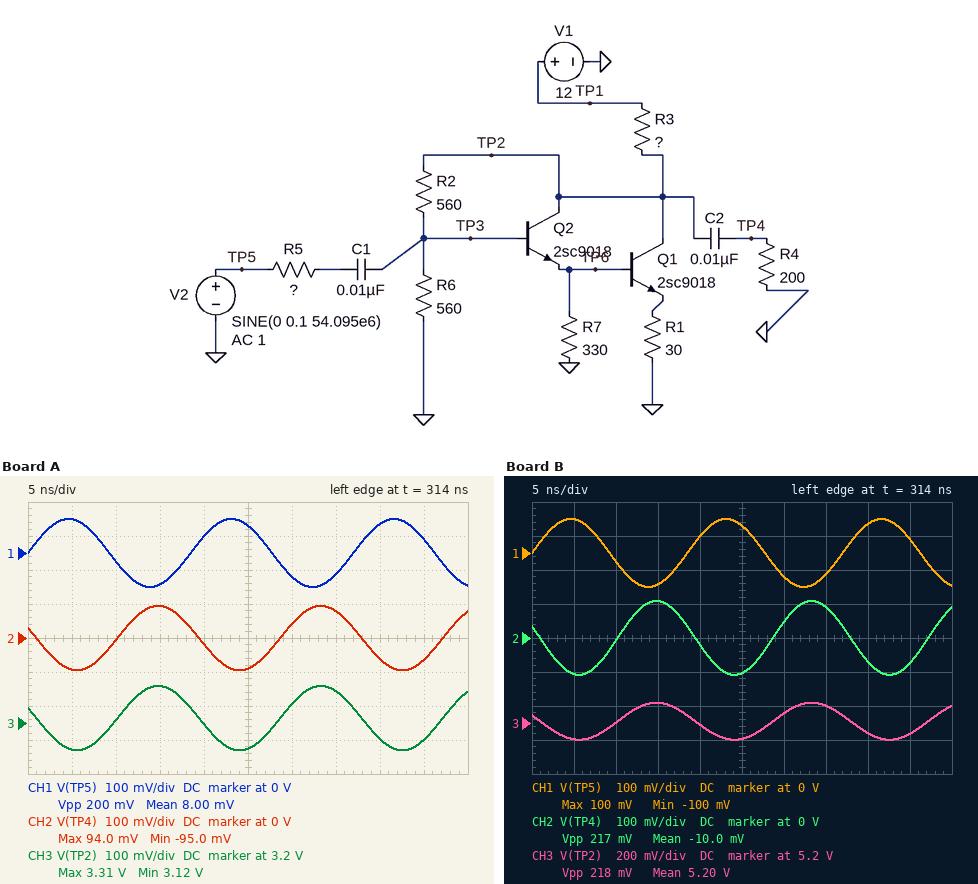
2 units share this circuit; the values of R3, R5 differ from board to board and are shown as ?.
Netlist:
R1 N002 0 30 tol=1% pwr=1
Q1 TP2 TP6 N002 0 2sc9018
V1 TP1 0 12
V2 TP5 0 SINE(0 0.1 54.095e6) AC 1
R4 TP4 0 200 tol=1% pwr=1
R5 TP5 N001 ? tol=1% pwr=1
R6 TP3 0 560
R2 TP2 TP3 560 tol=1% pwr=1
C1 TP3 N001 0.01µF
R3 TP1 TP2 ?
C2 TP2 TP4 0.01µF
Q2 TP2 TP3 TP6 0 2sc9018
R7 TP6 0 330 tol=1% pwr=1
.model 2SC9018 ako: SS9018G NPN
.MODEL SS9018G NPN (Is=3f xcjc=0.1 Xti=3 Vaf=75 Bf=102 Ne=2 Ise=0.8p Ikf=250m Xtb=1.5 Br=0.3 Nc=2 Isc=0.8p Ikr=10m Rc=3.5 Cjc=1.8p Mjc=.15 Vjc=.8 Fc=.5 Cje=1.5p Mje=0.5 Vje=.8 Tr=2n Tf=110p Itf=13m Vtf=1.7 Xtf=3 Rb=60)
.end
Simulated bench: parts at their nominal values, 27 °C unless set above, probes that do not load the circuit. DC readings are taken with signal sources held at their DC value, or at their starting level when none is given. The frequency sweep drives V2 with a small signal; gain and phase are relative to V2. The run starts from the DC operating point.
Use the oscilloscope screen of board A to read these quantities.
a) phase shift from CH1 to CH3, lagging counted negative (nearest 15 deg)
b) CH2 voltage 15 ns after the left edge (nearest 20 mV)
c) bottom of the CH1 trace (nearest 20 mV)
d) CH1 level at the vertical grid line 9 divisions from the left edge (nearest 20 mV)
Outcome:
165 deg
100 mV
-100 mV
40 mV
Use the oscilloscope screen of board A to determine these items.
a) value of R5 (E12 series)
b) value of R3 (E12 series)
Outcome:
270 Ω
820 Ω
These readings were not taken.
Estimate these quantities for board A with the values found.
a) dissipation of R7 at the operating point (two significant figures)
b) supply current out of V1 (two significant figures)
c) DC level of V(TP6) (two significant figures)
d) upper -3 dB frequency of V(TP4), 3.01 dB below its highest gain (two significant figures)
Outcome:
2.4 mW
11 mA
890 mV
270 MHz
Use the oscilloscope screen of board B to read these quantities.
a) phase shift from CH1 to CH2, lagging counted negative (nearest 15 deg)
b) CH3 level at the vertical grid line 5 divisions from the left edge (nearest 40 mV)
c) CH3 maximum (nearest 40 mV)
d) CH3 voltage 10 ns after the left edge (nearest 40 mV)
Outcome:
165 deg
5.12 V
5.32 V
5.20 V
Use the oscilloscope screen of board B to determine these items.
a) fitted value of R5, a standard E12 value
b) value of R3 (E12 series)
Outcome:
150 Ω
150 Ω
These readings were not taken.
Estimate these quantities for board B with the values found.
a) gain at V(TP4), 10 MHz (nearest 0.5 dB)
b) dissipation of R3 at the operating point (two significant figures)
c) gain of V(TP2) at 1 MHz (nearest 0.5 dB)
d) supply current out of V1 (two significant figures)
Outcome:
1.0 dB
310 mW
1.0 dB
45 mA
